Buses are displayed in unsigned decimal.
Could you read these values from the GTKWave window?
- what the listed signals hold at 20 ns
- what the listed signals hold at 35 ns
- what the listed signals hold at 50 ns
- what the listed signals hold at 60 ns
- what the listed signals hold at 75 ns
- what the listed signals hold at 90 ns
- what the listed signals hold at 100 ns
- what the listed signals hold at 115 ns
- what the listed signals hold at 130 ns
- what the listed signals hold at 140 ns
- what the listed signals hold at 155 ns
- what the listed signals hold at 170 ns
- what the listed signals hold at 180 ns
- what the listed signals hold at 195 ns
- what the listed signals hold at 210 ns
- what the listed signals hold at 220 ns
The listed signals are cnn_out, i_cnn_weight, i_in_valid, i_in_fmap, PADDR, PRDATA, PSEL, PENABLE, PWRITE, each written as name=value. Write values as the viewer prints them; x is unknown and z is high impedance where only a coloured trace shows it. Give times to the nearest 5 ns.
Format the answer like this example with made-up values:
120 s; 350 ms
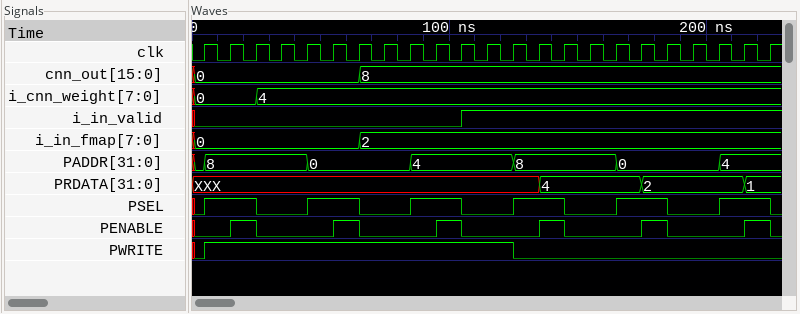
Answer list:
cnn_out=0, i_cnn_weight=0, i_in_valid=0, i_in_fmap=0, PADDR=8, PRDATA=XXX, PSEL=1, PENABLE=1, PWRITE=1; cnn_out=0, i_cnn_weight=4, i_in_valid=0, i_in_fmap=0, PADDR=8, PRDATA=XXX, PSEL=0, PENABLE=0, PWRITE=1; cnn_out=0, i_cnn_weight=4, i_in_valid=0, i_in_fmap=0, PADDR=0, PRDATA=XXX, PSEL=1, PENABLE=0, PWRITE=1; cnn_out=0, i_cnn_weight=4, i_in_valid=0, i_in_fmap=0, PADDR=0, PRDATA=XXX, PSEL=1, PENABLE=1, PWRITE=1; cnn_out=8, i_cnn_weight=4, i_in_valid=0, i_in_fmap=2, PADDR=0, PRDATA=XXX, PSEL=0, PENABLE=0, PWRITE=1; cnn_out=8, i_cnn_weight=4, i_in_valid=0, i_in_fmap=2, PADDR=4, PRDATA=XXX, PSEL=1, PENABLE=0, PWRITE=1; cnn_out=8, i_cnn_weight=4, i_in_valid=0, i_in_fmap=2, PADDR=4, PRDATA=XXX, PSEL=1, PENABLE=1, PWRITE=1; cnn_out=8, i_cnn_weight=4, i_in_valid=1, i_in_fmap=2, PADDR=4, PRDATA=XXX, PSEL=0, PENABLE=0, PWRITE=1; cnn_out=8, i_cnn_weight=4, i_in_valid=1, i_in_fmap=2, PADDR=8, PRDATA=XXX, PSEL=1, PENABLE=0, PWRITE=0; cnn_out=8, i_cnn_weight=4, i_in_valid=1, i_in_fmap=2, PADDR=8, PRDATA=4, PSEL=1, PENABLE=1, PWRITE=0; cnn_out=8, i_cnn_weight=4, i_in_valid=1, i_in_fmap=2, PADDR=8, PRDATA=4, PSEL=0, PENABLE=0, PWRITE=0; cnn_out=8, i_cnn_weight=4, i_in_valid=1, i_in_fmap=2, PADDR=0, PRDATA=4, PSEL=1, PENABLE=0, PWRITE=0; cnn_out=8, i_cnn_weight=4, i_in_valid=1, i_in_fmap=2, PADDR=0, PRDATA=2, PSEL=1, PENABLE=1, PWRITE=0; cnn_out=8, i_cnn_weight=4, i_in_valid=1, i_in_fmap=2, PADDR=0, PRDATA=2, PSEL=0, PENABLE=0, PWRITE=0; cnn_out=8, i_cnn_weight=4, i_in_valid=1, i_in_fmap=2, PADDR=4, PRDATA=2, PSEL=1, PENABLE=0, PWRITE=0; cnn_out=8, i_cnn_weight=4, i_in_valid=1, i_in_fmap=2, PADDR=4, PRDATA=1, PSEL=1, PENABLE=1, PWRITE=0
